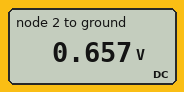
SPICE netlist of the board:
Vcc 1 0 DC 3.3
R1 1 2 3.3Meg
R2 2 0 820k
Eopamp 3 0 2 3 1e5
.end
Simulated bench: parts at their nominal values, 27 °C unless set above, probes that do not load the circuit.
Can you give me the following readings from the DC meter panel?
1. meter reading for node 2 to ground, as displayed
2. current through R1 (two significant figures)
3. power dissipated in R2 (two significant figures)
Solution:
0.657 V
800 nA
530 nW
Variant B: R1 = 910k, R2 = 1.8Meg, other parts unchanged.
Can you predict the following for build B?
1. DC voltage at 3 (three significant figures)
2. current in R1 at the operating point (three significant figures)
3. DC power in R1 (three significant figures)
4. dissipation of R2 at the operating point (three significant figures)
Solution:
2.19 V
1.22 µA
1.35 µW
2.67 µW
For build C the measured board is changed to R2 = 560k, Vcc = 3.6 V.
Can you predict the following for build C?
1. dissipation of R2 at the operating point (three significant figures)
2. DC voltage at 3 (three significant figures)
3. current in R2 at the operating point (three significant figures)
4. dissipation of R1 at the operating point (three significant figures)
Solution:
487 nW
522 mV
933 nA
2.87 µW
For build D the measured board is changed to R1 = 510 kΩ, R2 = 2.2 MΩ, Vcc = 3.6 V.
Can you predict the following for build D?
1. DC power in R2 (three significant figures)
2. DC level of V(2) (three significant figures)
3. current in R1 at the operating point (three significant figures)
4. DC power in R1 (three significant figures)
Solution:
3.88 µW
2.92 V
1.33 µA
900 nW
